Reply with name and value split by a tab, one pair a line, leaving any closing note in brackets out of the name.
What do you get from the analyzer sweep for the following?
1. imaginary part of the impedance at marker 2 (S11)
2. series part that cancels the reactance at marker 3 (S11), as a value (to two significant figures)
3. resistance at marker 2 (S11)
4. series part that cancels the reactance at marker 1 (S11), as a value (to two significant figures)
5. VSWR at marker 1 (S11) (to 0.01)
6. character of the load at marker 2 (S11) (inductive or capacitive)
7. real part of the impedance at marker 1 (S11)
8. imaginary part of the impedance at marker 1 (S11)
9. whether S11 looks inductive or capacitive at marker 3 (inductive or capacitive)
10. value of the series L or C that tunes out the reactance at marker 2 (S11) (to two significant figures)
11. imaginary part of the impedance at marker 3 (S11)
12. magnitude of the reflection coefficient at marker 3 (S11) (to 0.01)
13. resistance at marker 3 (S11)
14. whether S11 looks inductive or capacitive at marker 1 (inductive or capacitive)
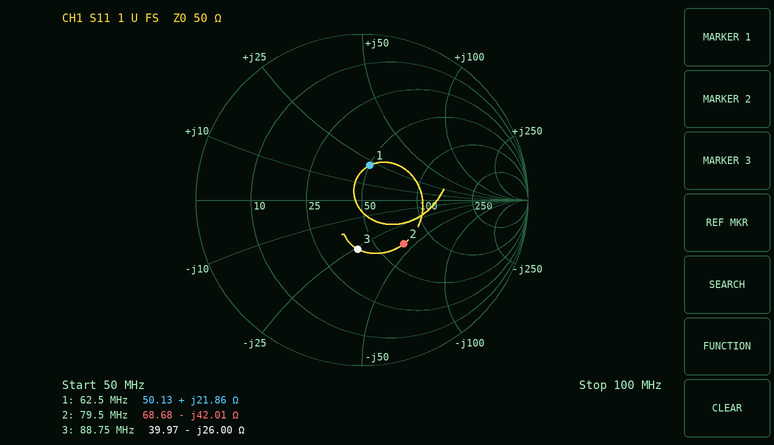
imaginary part of the impedance at marker 2	-42.01 Ω
series part that cancels the reactance at marker 3 (S11), as a value	47 nH
resistance at marker 2	68.68 Ω
series part that cancels the reactance at marker 1 (S11), as a value	120 pF
VSWR at marker 1 (S11)	1.54
character of the load at marker 2 (S11)	capacitive
real part of the impedance at marker 1	50.13 Ω
imaginary part of the impedance at marker 1	+21.86 Ω
whether S11 looks inductive or capacitive at marker 3	capacitive
value of the series L or C that tunes out the reactance at marker 2 (S11)	84 nH
imaginary part of the impedance at marker 3	-26.00 Ω
magnitude of the reflection coefficient at marker 3 (S11)	0.30
resistance at marker 3	39.97 Ω
whether S11 looks inductive or capacitive at marker 1	inductive
